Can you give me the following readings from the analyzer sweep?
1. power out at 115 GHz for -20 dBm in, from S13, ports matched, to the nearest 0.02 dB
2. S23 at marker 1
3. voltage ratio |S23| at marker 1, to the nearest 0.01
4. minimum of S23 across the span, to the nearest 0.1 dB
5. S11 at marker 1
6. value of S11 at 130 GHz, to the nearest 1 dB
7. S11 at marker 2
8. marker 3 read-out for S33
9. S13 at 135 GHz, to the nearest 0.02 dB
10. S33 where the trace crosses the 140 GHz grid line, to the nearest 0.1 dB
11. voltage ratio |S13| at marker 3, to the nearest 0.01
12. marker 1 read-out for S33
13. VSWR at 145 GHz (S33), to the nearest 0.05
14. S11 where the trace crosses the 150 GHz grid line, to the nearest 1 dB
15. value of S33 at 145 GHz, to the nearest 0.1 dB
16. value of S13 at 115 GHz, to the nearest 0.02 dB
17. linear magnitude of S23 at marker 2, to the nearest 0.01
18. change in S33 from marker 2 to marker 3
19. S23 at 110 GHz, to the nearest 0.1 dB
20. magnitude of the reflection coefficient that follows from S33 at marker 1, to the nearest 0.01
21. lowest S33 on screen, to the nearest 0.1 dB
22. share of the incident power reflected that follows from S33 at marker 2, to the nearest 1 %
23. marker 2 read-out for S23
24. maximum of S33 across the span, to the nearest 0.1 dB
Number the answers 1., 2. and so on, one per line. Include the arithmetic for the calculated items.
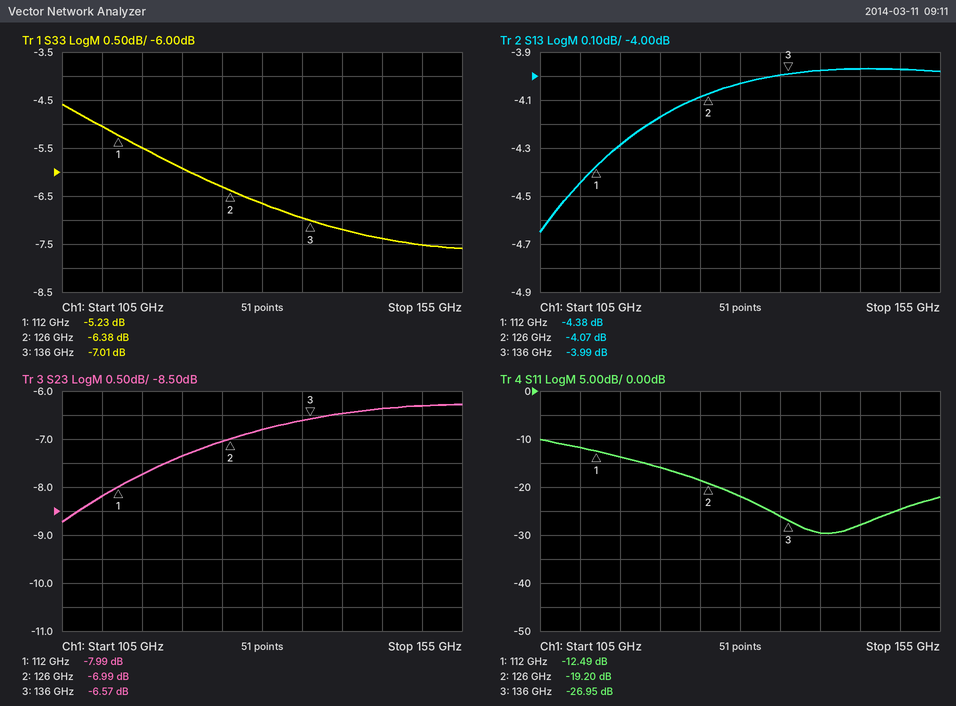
1. -20 dBm + (-4.28 dB) = -24.28 dBm
2. -7.99 dB
3. 10^(-7.99/20) ≈ 0.40
4. -8.7 dB
5. -12.49 dB
6. -22 dB
7. -19.20 dB
8. -7.01 dB
9. -4.00 dB
10. -7.2 dB
11. 10^(-3.99/20) ≈ 0.63
12. -5.23 dB
13. |Γ| = 10^(-7.4/20) = 0.4266; VSWR = (1 + 0.4266)/(1 − 0.4266) ≈ 2.49, so 2.50 to the nearest 0.05
14. -25 dB
15. -7.4 dB
16. -4.28 dB
17. 10^(-6.99/20) ≈ 0.45
18. -7.01 − (-6.38) = -0.63 dB
19. -8.2 dB
20. 10^(-5.23/20) ≈ 0.55
21. -7.6 dB
22. 10^(-6.38/10) ≈ 23 %
23. -6.99 dB
24. -4.6 dB
